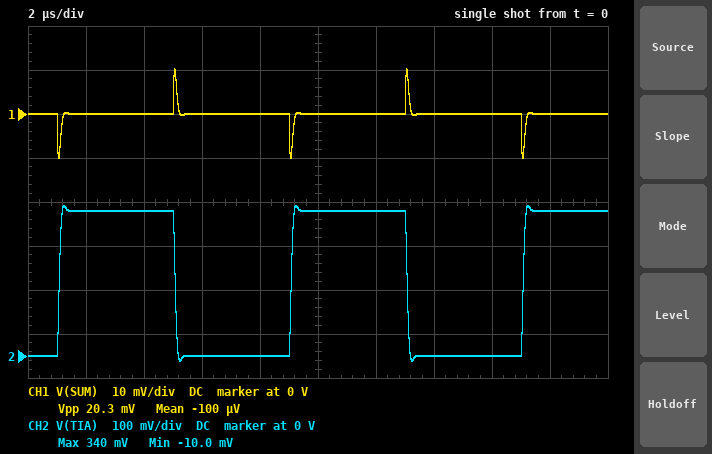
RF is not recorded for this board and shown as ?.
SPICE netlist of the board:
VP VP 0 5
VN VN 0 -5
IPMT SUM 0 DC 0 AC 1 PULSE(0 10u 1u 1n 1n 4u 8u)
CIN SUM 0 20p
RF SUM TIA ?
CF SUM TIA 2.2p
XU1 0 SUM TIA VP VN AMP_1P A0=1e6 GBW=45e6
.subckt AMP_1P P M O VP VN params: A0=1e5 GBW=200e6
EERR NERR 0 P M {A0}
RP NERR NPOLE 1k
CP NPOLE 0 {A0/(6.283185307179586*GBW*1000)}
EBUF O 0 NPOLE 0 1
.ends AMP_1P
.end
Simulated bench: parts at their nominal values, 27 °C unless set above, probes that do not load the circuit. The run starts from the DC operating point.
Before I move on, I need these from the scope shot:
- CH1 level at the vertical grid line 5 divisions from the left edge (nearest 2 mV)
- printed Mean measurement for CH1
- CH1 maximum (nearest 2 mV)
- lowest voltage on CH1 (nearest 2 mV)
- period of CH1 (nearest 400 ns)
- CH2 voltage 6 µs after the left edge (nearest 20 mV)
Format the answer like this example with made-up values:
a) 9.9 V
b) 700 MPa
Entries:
a) 0 V
b) -100 µV
c) 10 mV
d) -10 mV
e) 8.0 µs
f) 0 V
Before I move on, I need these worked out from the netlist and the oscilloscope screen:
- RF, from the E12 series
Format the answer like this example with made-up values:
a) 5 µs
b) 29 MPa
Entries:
a) 33 kΩ
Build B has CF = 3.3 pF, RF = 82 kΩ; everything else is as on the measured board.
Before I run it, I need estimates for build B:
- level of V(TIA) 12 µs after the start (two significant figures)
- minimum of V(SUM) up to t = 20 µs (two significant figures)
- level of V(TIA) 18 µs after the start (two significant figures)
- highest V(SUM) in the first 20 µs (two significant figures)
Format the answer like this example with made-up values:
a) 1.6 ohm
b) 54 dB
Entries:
a) 820 mV
b) -9.0 mV
c) 800 mV
d) 9.0 mV
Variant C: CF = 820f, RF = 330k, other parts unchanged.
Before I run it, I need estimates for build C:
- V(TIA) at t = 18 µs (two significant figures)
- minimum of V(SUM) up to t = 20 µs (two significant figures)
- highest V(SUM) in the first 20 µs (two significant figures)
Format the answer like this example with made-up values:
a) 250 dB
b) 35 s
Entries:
a) 3.3 V
b) -30 mV
c) 30 mV
